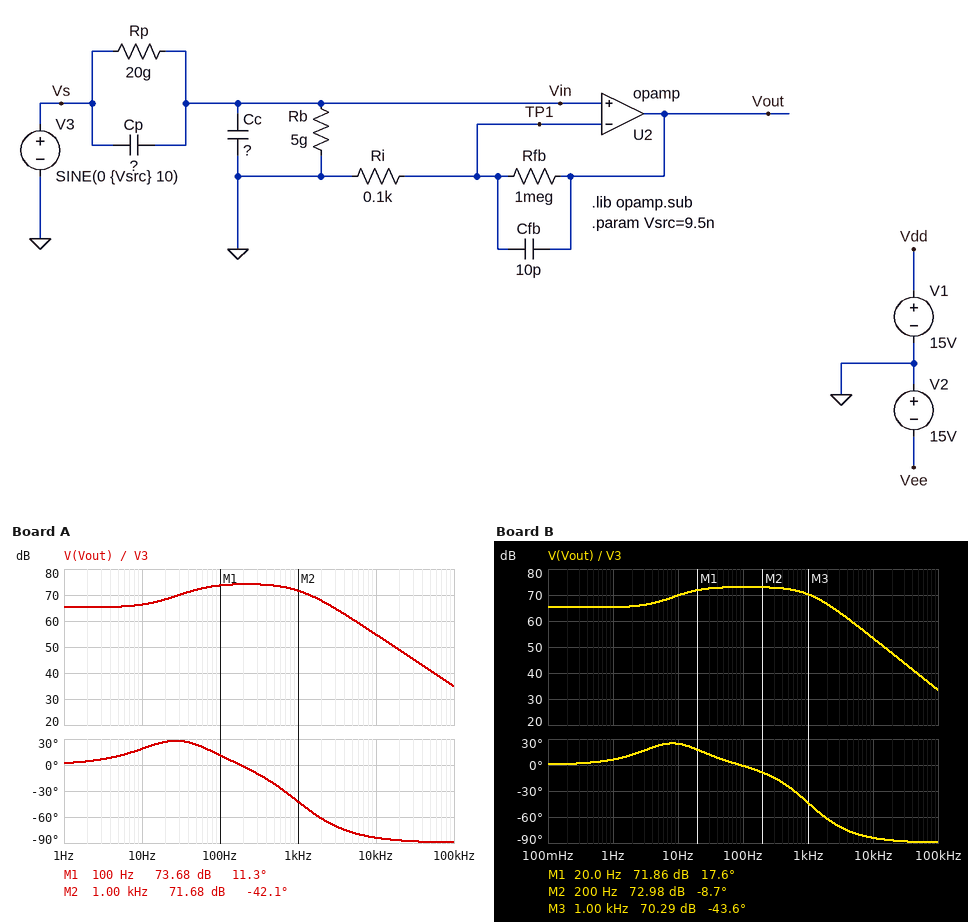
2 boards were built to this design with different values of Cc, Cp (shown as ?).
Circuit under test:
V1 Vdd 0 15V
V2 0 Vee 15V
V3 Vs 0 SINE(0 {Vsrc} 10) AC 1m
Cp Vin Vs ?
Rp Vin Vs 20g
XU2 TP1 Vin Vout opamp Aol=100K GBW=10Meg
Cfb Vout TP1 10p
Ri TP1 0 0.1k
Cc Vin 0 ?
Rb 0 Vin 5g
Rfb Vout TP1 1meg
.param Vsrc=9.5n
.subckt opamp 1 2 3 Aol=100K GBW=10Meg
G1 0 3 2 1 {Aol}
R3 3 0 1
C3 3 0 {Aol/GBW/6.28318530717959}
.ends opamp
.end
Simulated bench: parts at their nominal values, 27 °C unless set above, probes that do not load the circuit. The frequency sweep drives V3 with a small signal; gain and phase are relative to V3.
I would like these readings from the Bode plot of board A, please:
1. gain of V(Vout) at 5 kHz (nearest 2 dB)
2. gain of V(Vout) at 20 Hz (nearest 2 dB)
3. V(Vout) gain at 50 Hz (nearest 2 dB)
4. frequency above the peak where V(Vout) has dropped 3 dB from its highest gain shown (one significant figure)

60 dB
68 dB
72 dB
1 kHz
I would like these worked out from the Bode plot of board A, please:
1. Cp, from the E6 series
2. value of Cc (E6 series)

470 fF
330 fF
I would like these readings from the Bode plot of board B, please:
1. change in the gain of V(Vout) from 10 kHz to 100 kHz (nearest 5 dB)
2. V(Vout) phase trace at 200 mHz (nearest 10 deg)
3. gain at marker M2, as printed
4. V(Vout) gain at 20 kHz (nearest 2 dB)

-20 dB
0 deg
72.98 dB
48 dB
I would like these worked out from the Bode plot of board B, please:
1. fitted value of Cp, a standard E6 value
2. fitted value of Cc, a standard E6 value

1.5 pF
1.5 pF
